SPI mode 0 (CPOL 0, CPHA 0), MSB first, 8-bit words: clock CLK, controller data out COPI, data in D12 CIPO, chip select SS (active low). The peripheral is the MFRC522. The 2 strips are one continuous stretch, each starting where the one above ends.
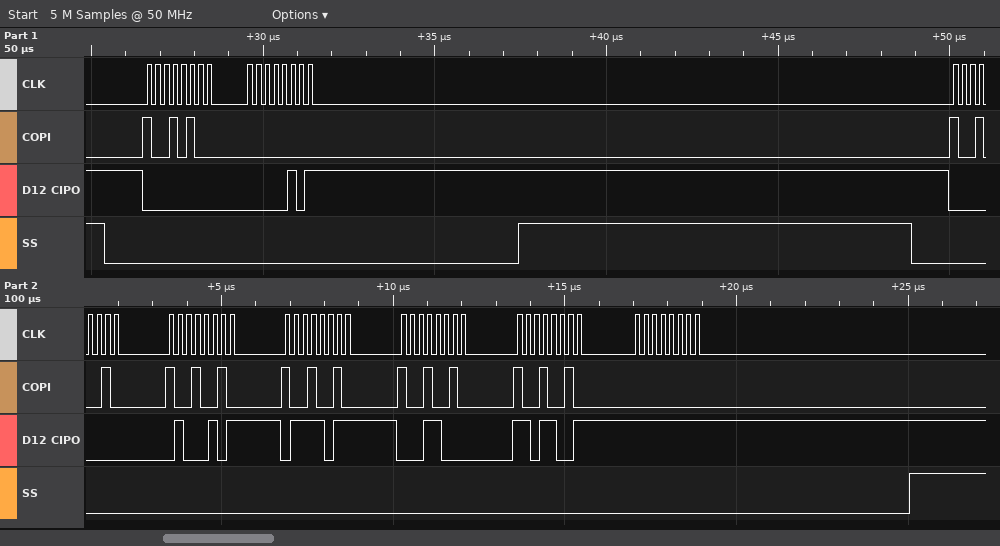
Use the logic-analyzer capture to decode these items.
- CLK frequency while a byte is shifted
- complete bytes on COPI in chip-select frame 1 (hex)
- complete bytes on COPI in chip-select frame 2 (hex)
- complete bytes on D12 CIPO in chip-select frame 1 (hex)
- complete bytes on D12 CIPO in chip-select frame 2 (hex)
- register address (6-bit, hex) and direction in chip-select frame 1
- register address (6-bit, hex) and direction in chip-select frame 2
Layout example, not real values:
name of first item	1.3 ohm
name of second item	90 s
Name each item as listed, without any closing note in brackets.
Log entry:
CLK frequency while a byte is shifted	4 MHz
complete bytes on COPI in chip-select frame 1	94 00
complete bytes on COPI in chip-select frame 2	92 92 92 92 92 00
complete bytes on D12 CIPO in chip-select frame 1	00 05
complete bytes on D12 CIPO in chip-select frame 2	00 45 7B 18 D9 FF
register address (6-bit, hex) and direction in chip-select frame 1	0x0A read
register address (6-bit, hex) and direction in chip-select frame 2	0x09 read
